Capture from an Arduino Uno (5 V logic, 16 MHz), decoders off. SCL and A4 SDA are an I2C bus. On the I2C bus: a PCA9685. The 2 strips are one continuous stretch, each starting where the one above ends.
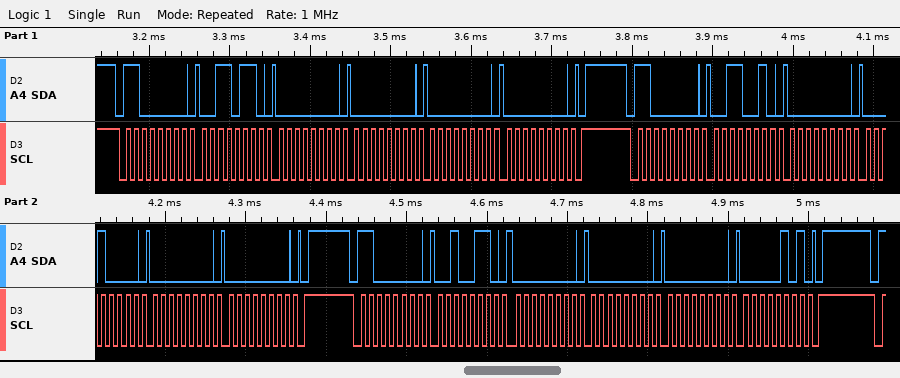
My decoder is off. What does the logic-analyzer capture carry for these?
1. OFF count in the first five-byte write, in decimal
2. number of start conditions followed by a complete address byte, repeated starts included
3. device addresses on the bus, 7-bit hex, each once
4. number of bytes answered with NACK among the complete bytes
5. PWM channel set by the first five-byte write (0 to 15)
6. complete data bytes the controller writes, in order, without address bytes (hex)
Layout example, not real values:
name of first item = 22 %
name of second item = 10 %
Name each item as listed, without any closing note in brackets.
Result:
OFF count in the first five-byte write, in decimal = 0
number of start conditions followed by a complete address byte, repeated starts included = 3
device addresses on the bus, 7-bit hex, each once = 0x60
number of bytes answered with NACK among the complete bytes = 0
PWM channel set by the first five-byte write = 12
complete data bytes the controller writes, in order, without address bytes = 36 00 00 00 00 32 00 10 00 00 26 00 00 00 05
